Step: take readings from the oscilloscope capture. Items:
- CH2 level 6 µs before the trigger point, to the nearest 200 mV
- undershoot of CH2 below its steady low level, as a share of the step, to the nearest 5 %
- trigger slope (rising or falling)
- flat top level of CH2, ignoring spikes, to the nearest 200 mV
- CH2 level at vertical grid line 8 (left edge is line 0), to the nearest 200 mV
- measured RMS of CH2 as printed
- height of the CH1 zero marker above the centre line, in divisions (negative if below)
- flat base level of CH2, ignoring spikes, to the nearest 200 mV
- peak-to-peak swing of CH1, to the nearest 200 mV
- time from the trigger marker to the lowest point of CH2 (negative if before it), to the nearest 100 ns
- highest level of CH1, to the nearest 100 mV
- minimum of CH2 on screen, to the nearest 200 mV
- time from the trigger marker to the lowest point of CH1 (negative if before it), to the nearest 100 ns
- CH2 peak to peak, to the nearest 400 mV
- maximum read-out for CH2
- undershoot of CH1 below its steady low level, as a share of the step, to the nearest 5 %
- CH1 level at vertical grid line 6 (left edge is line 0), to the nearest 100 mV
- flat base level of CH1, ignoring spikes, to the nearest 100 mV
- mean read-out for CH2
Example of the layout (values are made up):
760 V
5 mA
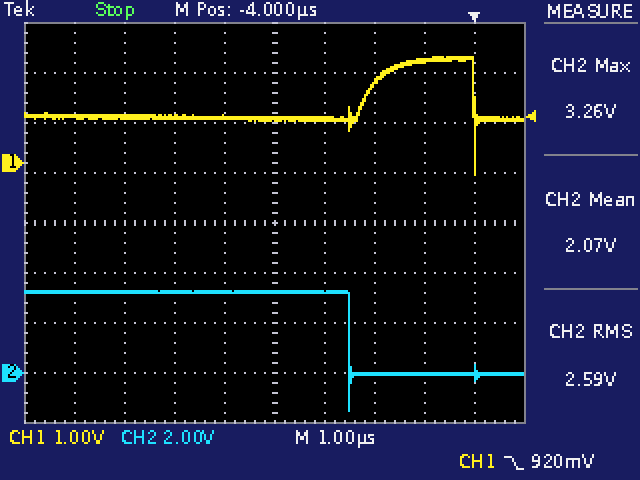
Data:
3.2 V
45 %
falling
3.2 V
0.0 V
2.59 V
+1.2 div
0.0 V
2.4 V
-2.5 µs
2.1 V
-1.6 V
0.0 µs
4.8 V
3.26 V
95 %
900 mV
900 mV
2.07 V
